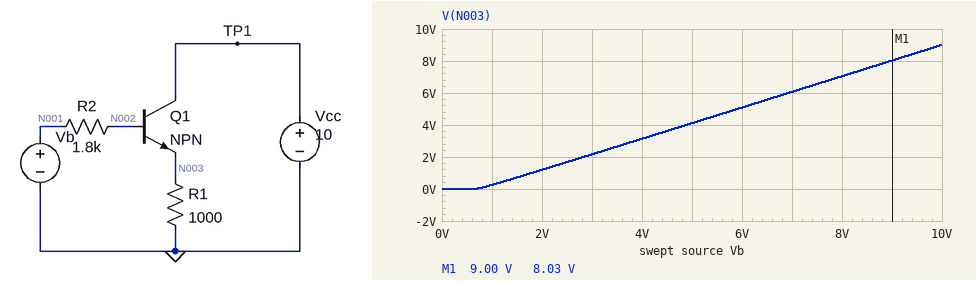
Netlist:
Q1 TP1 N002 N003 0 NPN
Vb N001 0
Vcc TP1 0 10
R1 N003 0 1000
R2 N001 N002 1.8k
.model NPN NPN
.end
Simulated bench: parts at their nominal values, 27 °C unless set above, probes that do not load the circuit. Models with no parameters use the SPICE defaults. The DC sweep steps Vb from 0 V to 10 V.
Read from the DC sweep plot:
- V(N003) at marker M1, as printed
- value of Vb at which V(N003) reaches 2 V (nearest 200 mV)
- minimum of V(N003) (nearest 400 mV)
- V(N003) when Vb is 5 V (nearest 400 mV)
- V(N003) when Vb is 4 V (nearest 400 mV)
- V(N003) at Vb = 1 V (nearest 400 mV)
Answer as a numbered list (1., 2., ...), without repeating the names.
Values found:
1. 8.03 V
2. 2.8 V
3. 0 V
4. 4.0 V
5. 3.2 V
6. 400 mV
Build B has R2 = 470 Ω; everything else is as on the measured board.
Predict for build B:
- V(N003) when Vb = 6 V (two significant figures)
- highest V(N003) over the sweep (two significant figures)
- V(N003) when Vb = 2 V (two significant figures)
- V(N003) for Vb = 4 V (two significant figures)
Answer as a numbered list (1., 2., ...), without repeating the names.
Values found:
1. 5.2 V
2. 9.1 V
3. 1.2 V
4. 3.2 V
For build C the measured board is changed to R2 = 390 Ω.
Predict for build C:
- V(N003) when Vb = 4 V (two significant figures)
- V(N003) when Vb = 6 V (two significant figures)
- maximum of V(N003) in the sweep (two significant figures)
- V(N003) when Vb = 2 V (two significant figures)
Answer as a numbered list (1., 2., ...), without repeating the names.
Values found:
1. 3.2 V
2. 5.2 V
3. 9.1 V
4. 1.2 V
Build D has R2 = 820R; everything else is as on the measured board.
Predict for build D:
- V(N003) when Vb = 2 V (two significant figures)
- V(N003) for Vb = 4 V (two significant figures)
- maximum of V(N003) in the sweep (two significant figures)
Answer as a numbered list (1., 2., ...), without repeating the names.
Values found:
1. 1.2 V
2. 3.2 V
3. 9.1 V
